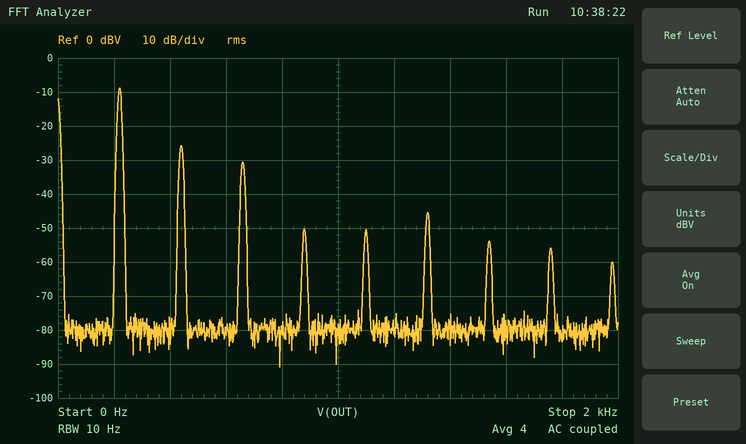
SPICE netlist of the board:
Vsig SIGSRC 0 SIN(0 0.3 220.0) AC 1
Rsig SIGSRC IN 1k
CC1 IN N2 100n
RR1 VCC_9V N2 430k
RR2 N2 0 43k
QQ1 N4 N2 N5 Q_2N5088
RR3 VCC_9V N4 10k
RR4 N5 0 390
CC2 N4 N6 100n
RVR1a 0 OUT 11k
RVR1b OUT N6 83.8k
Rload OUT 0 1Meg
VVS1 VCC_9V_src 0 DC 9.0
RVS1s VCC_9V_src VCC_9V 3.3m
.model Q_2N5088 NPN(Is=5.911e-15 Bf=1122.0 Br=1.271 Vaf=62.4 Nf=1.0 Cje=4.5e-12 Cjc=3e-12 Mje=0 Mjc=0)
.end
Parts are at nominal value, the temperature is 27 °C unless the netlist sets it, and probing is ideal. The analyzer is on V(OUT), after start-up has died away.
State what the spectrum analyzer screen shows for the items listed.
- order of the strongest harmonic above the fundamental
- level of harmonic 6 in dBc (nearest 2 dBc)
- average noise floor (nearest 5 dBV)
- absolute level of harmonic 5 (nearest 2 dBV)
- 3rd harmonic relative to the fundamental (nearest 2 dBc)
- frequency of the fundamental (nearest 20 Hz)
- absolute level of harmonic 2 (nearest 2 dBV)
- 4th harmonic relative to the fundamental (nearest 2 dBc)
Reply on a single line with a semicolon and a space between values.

2; -36 dBc; -80 dBV; -50 dBV; -22 dBc; 220 Hz; -26 dBV; -42 dBc
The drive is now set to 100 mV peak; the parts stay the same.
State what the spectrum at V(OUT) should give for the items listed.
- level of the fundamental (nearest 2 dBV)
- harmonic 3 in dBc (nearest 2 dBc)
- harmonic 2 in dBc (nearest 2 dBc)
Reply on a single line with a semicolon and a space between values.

-16 dBV; -52 dBc; -34 dBc
